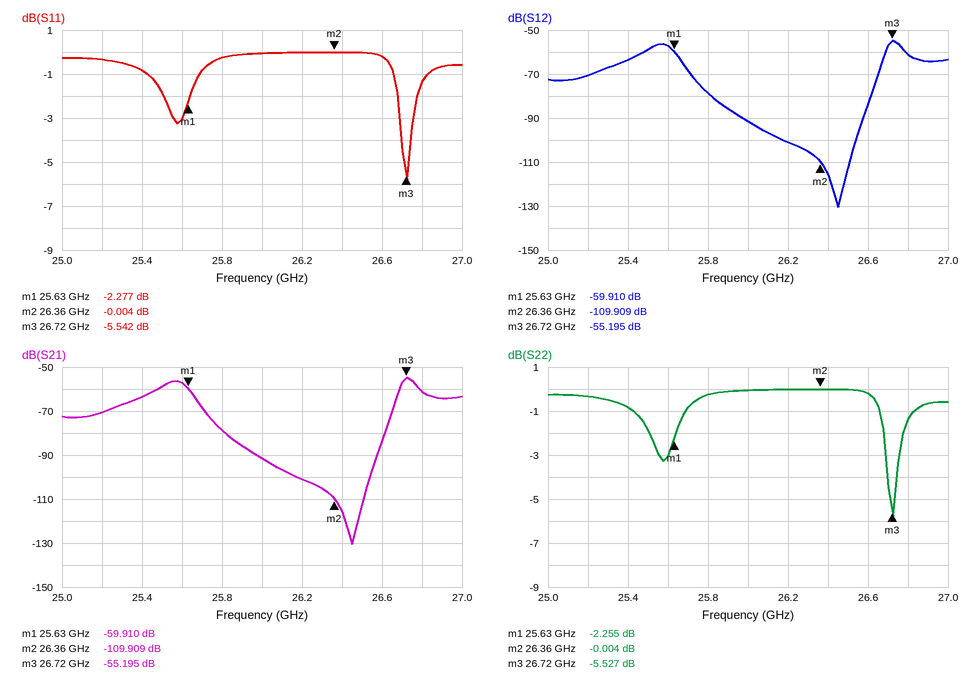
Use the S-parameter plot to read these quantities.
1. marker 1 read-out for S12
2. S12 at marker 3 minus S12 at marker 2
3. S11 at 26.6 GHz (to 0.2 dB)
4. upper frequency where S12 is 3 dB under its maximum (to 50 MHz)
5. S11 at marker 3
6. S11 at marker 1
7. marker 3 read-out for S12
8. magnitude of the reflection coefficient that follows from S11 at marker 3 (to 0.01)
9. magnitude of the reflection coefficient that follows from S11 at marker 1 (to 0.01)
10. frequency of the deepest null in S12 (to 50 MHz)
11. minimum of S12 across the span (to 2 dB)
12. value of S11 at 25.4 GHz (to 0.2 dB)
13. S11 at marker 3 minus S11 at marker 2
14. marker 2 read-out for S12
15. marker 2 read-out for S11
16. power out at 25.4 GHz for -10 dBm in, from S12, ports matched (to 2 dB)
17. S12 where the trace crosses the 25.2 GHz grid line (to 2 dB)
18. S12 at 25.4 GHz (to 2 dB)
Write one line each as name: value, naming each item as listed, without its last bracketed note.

marker 1 read-out for S12: -59.910 dB
S12 at marker 3 minus S12 at marker 2: 54.714 dB
S11 at 26.6 GHz: -0.2 dB
upper frequency where S12 is 3 dB under its maximum: 26.75 GHz
S11 at marker 3: -5.542 dB
S11 at marker 1: -2.277 dB
marker 3 read-out for S12: -55.195 dB
magnitude of the reflection coefficient that follows from S11 at marker 3: 0.53
magnitude of the reflection coefficient that follows from S11 at marker 1: 0.77
frequency of the deepest null in S12: 26.45 GHz
minimum of S12 across the span: -130 dB
value of S11 at 25.4 GHz: -0.8 dB
S11 at marker 3 minus S11 at marker 2: -5.538 dB
marker 2 read-out for S12: -109.909 dB
marker 2 read-out for S11: -0.004 dB
power out at 25.4 GHz for -10 dBm in, from S12, ports matched: -74 dBm
S12 where the trace crosses the 25.2 GHz grid line: -70 dB
S12 at 25.4 GHz: -64 dB
